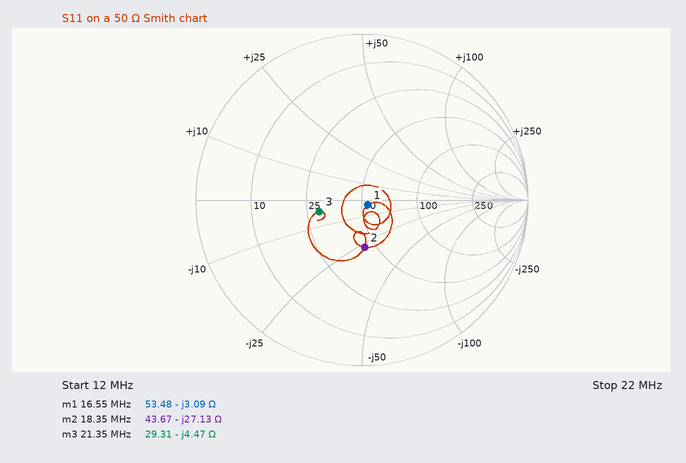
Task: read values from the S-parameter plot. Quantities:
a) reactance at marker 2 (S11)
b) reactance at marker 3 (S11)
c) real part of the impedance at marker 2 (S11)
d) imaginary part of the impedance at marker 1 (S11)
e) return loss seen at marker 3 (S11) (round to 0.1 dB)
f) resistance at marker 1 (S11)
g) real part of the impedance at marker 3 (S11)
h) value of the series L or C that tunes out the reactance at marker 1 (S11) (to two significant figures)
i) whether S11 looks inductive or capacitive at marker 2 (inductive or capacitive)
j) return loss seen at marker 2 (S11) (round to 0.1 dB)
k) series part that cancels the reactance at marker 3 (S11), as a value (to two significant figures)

-27.13 Ω
-4.47 Ω
43.67 Ω
-3.09 Ω
11.5 dB
53.48 Ω
29.31 Ω
30 nH
capacitive
10.9 dB
33 nH
